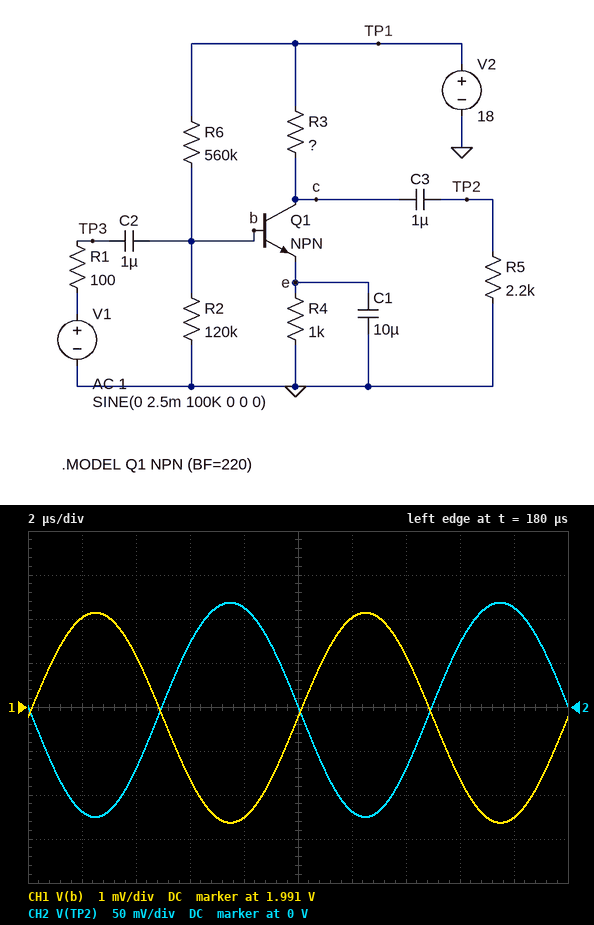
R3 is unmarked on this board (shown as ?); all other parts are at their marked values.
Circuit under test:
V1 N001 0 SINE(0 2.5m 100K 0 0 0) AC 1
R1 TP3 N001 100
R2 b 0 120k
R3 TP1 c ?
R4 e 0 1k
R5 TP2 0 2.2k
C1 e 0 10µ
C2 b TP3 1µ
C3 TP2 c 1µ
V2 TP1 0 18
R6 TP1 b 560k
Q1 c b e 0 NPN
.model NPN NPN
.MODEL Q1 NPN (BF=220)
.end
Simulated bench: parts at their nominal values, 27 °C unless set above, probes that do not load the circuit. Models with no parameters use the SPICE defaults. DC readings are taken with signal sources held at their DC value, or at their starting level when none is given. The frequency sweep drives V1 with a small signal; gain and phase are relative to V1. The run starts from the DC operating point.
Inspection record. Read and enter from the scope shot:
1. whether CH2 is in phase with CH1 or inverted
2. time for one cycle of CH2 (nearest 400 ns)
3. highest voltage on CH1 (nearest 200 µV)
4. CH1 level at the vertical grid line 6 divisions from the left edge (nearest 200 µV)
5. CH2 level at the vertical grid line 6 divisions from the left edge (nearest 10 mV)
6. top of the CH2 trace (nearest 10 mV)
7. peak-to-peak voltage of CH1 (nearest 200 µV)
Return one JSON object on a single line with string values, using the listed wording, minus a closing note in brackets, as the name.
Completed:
{"whether CH2 is in phase with CH1 or inverted": "inverted", "time for one cycle of CH2": "10.0 µs", "highest voltage on CH1": "1.9932 V", "CH1 level at the vertical grid line 6 divisions from the left edge": "1.9930 V", "CH2 level at the vertical grid line 6 divisions from the left edge": "-120 mV", "top of the CH2 trace": "120 mV", "peak-to-peak voltage of CH1": "4.8 mV"}
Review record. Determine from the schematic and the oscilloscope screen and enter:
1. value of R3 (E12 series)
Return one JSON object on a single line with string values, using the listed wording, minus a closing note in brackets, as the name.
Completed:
{"value of R3": "2.2 kΩ"}
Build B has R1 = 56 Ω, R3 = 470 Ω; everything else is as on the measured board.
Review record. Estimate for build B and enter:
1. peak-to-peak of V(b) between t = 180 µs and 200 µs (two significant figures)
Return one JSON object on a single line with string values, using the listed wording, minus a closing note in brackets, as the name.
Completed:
{"peak-to-peak of V(b) between t = 180 µs and 200 µs": "4.9 mV"}
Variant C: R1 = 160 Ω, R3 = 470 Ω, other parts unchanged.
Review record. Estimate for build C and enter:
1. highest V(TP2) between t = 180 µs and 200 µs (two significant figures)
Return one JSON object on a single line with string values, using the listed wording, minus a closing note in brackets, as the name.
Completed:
{"highest V(TP2) between t = 180 µs and 200 µs": "41 mV"}
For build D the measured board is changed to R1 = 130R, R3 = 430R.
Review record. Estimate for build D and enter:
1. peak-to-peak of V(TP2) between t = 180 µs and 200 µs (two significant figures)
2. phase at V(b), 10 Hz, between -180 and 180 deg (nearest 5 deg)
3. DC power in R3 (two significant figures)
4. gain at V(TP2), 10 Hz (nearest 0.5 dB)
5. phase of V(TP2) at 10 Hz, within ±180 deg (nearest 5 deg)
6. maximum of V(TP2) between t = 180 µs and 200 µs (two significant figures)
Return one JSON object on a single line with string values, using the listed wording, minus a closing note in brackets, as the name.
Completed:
{"peak-to-peak of V(TP2) between t = 180 µs and 200 µs": "79 mV", "phase at V(b), 10 Hz, between -180 and 180 deg": "15 deg", "DC power in R3": "620 µW", "gain at V(TP2), 10 Hz": "-24.5 dB", "phase of V(TP2) at 10 Hz, within ±180 deg": "-50 deg", "maximum of V(TP2) between t = 180 µs and 200 µs": "38 mV"}
